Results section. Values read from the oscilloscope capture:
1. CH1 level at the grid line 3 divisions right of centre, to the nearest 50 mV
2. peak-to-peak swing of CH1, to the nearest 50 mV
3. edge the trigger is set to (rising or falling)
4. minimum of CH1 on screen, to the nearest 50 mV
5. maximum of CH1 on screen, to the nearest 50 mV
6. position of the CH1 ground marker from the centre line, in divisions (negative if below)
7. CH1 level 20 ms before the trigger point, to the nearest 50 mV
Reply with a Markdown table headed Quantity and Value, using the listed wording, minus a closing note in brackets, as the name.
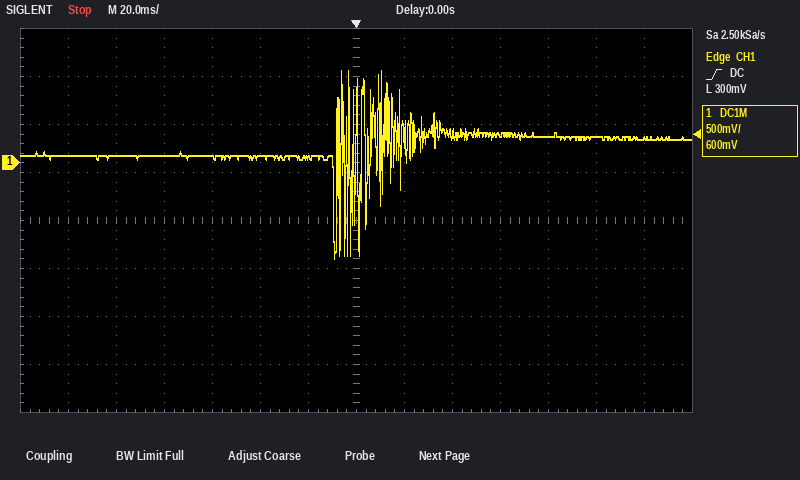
| Quantity | Value |
|---|---|
| CH1 level at the grid line 3 divisions right of centre, to the nearest 50 mV | 300 mV |
| peak-to-peak swing of CH1, to the nearest 50 mV | 1.95 V |
| edge the trigger is set to | rising |
| minimum of CH1 on screen, to the nearest 50 mV | -1.00 V |
| maximum of CH1 on screen, to the nearest 50 mV | 950 mV |
| position of the CH1 ground marker from the centre line, in divisions | +1.2 div |
| CH1 level 20 ms before the trigger point, to the nearest 50 mV | 50 mV |
